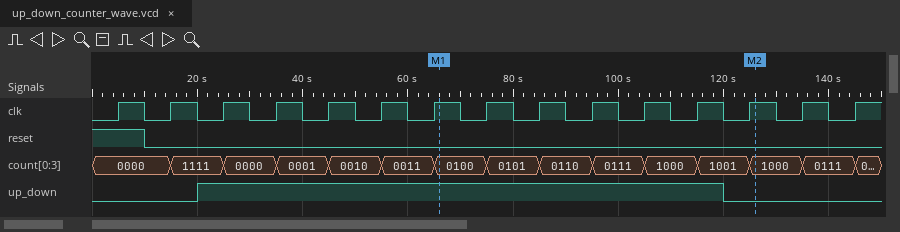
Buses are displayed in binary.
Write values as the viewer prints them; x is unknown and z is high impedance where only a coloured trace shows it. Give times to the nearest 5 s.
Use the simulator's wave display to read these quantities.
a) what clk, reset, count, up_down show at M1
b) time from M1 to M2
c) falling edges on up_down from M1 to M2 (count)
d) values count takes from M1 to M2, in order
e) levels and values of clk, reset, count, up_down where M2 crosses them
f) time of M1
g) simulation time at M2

clk=1, reset=0, count=0100, up_down=1
60 s
1
0100, 0101, 0110, 0111, 1000, 1001, 1000
clk=1, reset=0, count=1000, up_down=0
65 s
125 s
